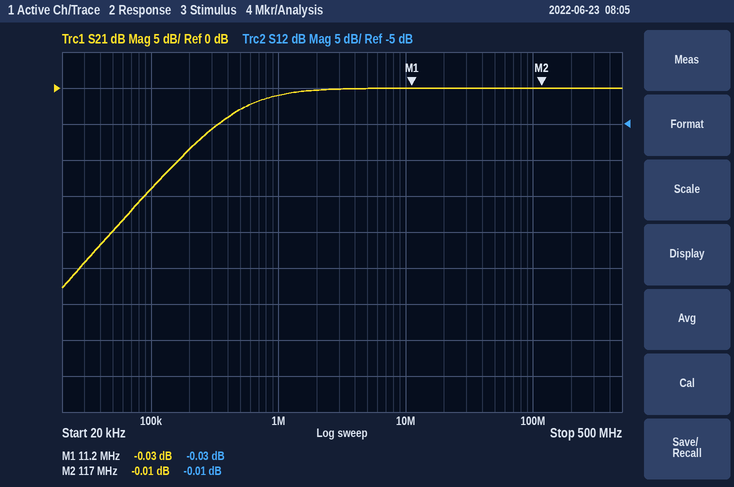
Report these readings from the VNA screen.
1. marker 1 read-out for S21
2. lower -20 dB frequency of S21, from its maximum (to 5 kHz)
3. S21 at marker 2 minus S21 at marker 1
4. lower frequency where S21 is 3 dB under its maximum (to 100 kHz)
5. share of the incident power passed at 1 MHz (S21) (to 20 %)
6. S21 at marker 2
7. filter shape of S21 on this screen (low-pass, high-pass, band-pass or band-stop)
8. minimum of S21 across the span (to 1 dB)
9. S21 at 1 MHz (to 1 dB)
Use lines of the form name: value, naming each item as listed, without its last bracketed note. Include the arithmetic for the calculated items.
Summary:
marker 1 read-out for S21: -0.03 dB
lower -20 dB frequency of S21, from its maximum: 50 kHz
S21 at marker 2 minus S21 at marker 1: -0.01 − (-0.03) = 0.02 dB
lower frequency where S21 is 3 dB under its maximum: 500 kHz
share of the incident power passed at 1 MHz (S21): 10^(-1/10) ≈ 79.4 %, so 80 % to the nearest 20 %
S21 at marker 2: -0.01 dB
filter shape of S21 on this screen: high-pass
minimum of S21 across the span: -28 dB
S21 at 1 MHz: -1 dB
